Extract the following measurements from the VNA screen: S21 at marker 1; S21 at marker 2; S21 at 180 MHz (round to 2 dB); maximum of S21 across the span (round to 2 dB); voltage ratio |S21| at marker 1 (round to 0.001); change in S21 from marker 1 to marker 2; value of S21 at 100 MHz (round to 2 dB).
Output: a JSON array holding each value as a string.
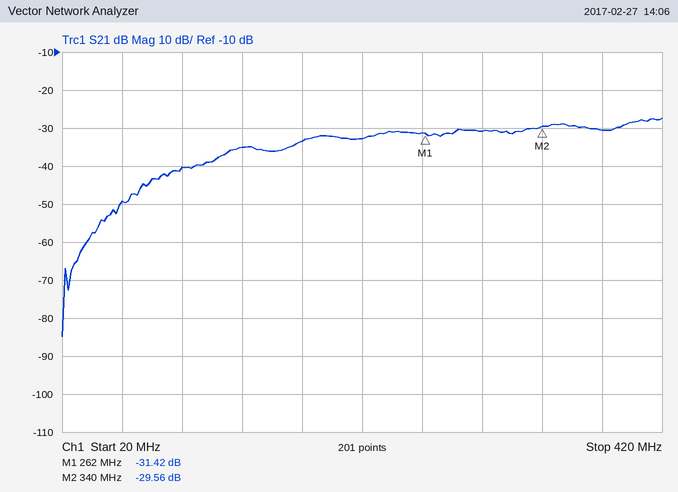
["-31.42 dB", "-29.56 dB", "-34 dB", "-28 dB", "0.027", "1.86 dB", "-40 dB"]
